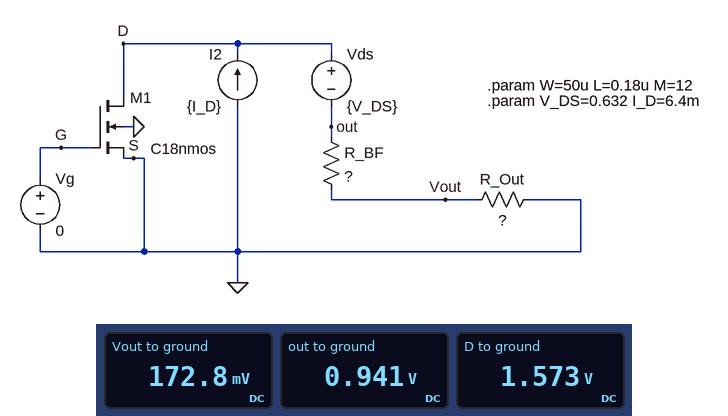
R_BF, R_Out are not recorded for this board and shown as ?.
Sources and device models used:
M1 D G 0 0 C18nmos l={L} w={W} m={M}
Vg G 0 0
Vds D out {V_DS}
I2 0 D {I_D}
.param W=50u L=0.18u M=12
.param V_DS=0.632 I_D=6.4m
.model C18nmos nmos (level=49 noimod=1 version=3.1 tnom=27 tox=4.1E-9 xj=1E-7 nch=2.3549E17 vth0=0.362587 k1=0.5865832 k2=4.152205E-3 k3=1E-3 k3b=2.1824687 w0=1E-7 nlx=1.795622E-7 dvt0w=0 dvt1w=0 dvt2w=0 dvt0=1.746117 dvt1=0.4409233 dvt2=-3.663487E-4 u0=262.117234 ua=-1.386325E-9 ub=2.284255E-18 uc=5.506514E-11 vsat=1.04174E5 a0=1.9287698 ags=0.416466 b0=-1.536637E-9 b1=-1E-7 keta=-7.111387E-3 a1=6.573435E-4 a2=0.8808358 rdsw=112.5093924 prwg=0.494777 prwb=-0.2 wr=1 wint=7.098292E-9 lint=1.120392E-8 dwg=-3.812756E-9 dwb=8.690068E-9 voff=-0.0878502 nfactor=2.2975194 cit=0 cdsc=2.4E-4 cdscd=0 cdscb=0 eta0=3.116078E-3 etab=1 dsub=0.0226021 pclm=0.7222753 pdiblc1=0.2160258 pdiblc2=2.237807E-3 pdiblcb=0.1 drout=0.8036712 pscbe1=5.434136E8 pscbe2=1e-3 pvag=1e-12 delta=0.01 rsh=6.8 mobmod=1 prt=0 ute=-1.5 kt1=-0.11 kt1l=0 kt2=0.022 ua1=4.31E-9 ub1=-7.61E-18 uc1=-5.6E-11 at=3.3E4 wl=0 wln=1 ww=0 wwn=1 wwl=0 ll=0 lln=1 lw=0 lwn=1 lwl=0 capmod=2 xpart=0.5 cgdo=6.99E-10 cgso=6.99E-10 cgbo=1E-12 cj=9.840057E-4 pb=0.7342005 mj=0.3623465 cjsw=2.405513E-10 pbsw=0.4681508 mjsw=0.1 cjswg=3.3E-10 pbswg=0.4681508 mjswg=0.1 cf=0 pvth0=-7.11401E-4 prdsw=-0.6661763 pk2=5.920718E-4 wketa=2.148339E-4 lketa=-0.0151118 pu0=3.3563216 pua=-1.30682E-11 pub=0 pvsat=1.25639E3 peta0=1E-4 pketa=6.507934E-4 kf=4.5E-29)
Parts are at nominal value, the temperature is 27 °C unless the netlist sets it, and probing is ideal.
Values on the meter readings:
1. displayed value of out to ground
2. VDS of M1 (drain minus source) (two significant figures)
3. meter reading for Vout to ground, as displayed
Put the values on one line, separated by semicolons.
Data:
0.941 V; 1.6 V; 172.8 mV
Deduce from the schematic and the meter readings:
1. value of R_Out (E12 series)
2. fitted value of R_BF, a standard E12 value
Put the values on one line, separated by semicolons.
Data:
27 Ω; 120 Ω
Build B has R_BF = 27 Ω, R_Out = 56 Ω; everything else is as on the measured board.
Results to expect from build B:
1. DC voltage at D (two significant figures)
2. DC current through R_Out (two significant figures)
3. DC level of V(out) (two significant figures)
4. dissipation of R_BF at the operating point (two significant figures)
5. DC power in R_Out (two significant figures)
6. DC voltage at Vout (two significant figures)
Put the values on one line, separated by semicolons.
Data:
1.2 V; 6.4 mA; 530 mV; 1.1 mW; 2.3 mW; 360 mV
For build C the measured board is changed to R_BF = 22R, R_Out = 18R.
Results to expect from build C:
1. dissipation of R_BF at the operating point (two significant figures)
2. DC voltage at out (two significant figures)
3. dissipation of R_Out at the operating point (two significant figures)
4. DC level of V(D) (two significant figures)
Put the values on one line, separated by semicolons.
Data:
900 µW; 260 mV; 740 µW; 890 mV
